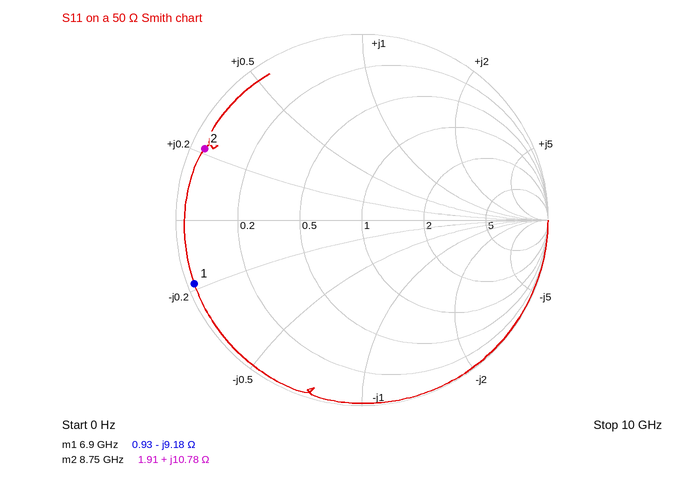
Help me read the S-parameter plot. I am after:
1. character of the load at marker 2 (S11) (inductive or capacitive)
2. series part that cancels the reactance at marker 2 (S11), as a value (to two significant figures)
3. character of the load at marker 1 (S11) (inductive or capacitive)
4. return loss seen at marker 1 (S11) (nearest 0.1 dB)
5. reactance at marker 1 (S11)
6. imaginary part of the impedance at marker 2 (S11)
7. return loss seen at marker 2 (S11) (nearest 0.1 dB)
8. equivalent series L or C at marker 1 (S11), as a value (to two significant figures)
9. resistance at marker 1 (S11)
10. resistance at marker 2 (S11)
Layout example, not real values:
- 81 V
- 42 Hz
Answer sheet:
- inductive
- 1.7 pF
- capacitive
- 0.3 dB
- -9.18 Ω
- +10.78 Ω
- 0.6 dB
- 2.5 pF
- 0.93 Ω
- 1.91 Ω
